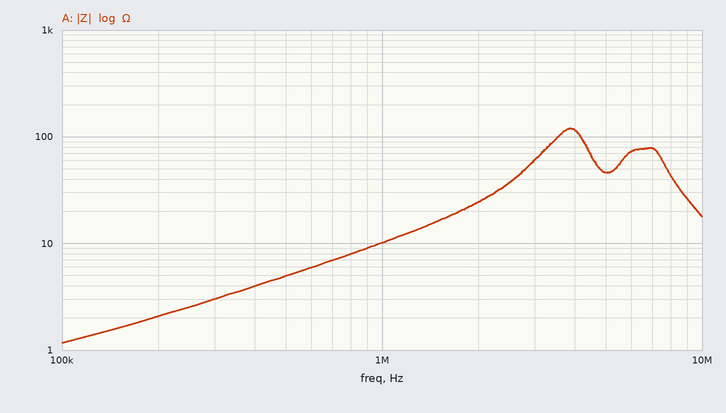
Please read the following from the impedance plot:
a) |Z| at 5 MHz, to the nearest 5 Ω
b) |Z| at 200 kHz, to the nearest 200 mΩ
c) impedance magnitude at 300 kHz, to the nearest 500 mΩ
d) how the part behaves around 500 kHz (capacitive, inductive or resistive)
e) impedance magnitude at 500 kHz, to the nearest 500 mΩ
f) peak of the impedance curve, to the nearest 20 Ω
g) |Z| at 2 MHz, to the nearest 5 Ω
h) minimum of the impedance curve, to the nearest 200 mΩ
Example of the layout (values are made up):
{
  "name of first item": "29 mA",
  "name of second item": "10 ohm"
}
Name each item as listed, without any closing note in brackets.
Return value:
{
  "|Z| at 5 MHz, to the nearest 5 Ω": "45 Ω",
  "|Z| at 200 kHz, to the nearest 200 mΩ": "2.0 Ω",
  "impedance magnitude at 300 kHz, to the nearest 500 mΩ": "3.0 Ω",
  "how the part behaves around 500 kHz": "inductive",
  "impedance magnitude at 500 kHz, to the nearest 500 mΩ": "5.0 Ω",
  "peak of the impedance curve, to the nearest 20 Ω": "120 Ω",
  "|Z| at 2 MHz, to the nearest 5 Ω": "25 Ω",
  "minimum of the impedance curve, to the nearest 200 mΩ": "1.2 Ω"
}
